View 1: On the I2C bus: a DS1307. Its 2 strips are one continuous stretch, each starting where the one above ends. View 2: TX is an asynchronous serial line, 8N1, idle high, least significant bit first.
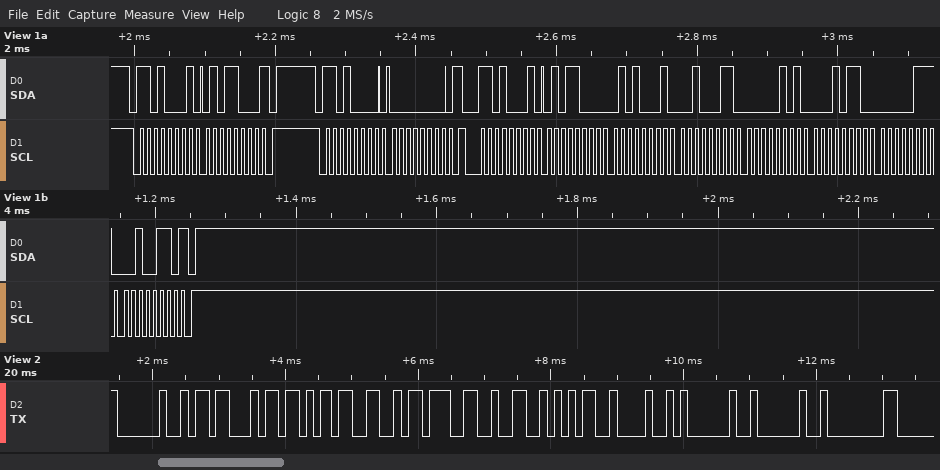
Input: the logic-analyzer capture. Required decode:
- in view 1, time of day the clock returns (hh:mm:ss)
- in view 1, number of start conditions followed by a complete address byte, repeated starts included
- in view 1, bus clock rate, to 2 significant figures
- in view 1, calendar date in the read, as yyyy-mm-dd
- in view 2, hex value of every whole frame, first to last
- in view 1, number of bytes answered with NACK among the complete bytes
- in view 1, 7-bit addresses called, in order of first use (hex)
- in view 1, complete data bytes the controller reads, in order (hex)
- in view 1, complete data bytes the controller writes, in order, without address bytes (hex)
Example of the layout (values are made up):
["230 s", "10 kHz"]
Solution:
["23:51:58", "3", "100 kHz", "2026-07-16", "20 1B 5B 33 3B 32 35 48 20 20 80", "2", "0x68", "58 58 51 23 05 16 07 26", "00"]
